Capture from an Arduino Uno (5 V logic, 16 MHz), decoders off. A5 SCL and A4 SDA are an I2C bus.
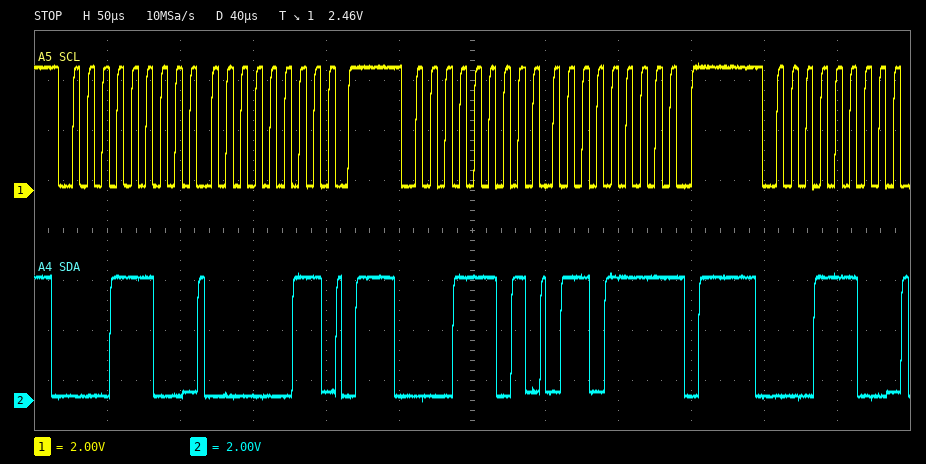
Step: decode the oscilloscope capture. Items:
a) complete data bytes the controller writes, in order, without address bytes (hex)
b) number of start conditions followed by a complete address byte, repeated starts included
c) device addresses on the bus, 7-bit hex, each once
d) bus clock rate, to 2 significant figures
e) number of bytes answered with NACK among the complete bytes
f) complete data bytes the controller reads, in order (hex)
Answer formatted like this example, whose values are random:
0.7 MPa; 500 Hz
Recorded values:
03; 3; 0x0E; 100 kHz; 1; 6F
